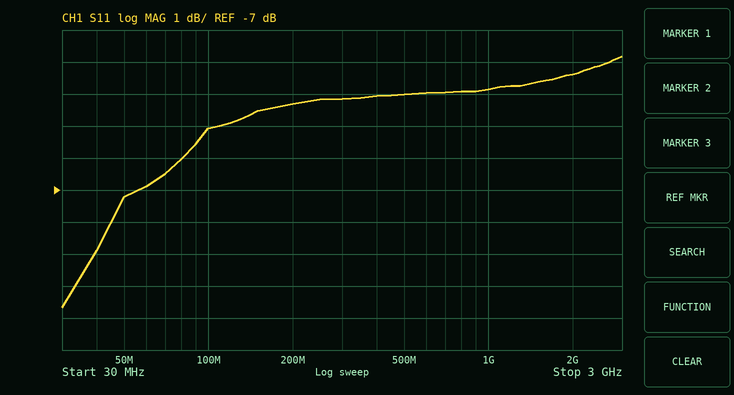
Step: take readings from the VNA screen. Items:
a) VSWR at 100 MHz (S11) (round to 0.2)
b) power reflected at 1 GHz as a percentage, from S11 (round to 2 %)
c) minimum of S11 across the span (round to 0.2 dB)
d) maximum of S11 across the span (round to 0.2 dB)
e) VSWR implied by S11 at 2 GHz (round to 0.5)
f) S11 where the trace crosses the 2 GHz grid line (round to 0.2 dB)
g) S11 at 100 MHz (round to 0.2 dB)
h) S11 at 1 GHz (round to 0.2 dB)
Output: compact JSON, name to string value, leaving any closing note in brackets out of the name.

{"VSWR at 100 MHz (S11)": "3.6", "power reflected at 1 GHz as a percentage, from S11": "42 %", "minimum of S11 across the span": "-10.6 dB", "maximum of S11 across the span": "-2.8 dB", "VSWR implied by S11 at 2 GHz": "5.0", "S11 where the trace crosses the 2 GHz grid line": "-3.4 dB", "S11 at 100 MHz": "-5.0 dB", "S11 at 1 GHz": "-3.8 dB"}
